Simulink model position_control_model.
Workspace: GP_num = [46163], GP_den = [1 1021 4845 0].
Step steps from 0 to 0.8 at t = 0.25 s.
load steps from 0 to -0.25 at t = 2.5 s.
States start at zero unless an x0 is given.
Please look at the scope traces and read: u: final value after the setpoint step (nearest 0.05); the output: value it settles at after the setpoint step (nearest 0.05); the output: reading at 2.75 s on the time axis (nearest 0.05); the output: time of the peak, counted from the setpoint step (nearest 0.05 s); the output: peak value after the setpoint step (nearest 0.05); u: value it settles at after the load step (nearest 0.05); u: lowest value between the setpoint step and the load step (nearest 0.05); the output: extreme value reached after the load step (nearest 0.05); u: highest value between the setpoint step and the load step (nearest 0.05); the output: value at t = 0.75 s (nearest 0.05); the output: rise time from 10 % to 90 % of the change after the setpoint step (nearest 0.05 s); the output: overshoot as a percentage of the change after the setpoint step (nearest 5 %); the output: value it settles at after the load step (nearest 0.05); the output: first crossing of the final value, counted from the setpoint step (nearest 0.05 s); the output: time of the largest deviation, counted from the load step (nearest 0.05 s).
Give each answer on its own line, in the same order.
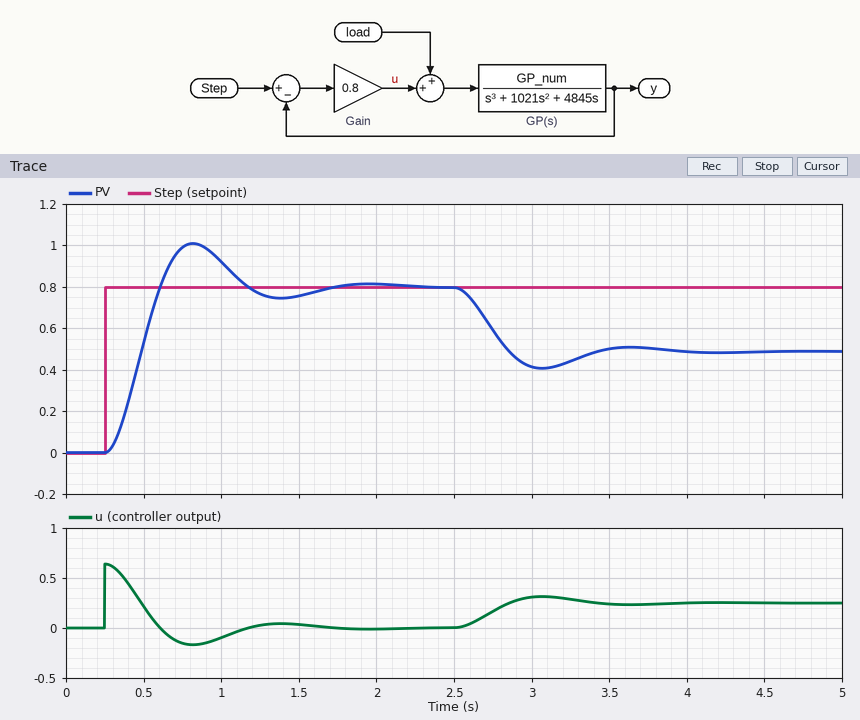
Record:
0.00
0.80
0.60
0.55 s
1.00
0.25
-0.15
0.40
0.65
1.00
0.25 s
25 %
0.50
0.35 s
0.55 s
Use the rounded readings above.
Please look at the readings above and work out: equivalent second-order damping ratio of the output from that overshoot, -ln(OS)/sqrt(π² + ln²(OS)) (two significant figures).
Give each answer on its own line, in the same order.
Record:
0.40
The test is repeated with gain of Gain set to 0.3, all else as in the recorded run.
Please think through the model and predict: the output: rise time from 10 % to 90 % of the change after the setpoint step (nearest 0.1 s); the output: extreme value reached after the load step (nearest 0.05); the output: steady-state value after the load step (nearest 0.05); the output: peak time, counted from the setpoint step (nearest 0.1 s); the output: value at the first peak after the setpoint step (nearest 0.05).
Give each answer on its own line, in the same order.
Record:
0.5 s
-0.10
-0.05
1.1 s
0.85
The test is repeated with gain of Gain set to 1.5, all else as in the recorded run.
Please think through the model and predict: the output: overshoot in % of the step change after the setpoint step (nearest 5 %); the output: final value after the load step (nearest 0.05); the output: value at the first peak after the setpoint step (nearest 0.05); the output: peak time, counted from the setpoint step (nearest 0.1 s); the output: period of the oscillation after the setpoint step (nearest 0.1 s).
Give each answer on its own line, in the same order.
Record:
40 %
0.65
1.10
0.4 s
0.8 s
